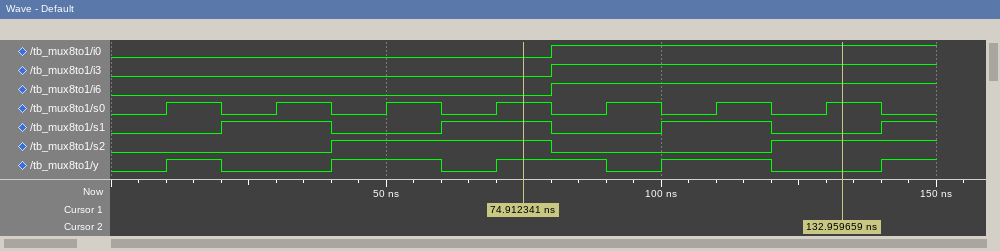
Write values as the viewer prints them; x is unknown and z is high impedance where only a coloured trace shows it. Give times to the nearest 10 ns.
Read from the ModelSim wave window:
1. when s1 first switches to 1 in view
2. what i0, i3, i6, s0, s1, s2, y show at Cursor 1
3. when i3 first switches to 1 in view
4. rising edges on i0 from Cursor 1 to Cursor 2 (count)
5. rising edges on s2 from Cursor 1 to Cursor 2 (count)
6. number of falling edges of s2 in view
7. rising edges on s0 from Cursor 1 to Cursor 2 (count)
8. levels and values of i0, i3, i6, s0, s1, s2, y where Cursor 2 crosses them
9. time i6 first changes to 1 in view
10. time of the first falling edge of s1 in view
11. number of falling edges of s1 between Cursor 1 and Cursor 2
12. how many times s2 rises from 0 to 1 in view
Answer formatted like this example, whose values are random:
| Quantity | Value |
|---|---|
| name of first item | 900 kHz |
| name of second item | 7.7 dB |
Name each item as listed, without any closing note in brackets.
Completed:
| Quantity | Value |
|---|---|
| when s1 first switches to 1 in view | 20 ns |
| what i0, i3, i6, s0, s1, s2, y show at Cursor 1 | i0=0, i3=0, i6=0, s0=1, s1=1, s2=1, y=1 |
| when i3 first switches to 1 in view | 80 ns |
| rising edges on i0 from Cursor 1 to Cursor 2 | 1 |
| rising edges on s2 from Cursor 1 to Cursor 2 | 1 |
| number of falling edges of s2 in view | 1 |
| rising edges on s0 from Cursor 1 to Cursor 2 | 3 |
| levels and values of i0, i3, i6, s0, s1, s2, y where Cursor 2 crosses them | i0=1, i3=1, i6=1, s0=1, s1=0, s2=1, y=0 |
| time i6 first changes to 1 in view | 80 ns |
| time of the first falling edge of s1 in view | 40 ns |
| number of falling edges of s1 between Cursor 1 and Cursor 2 | 2 |
| how many times s2 rises from 0 to 1 in view | 2 |
